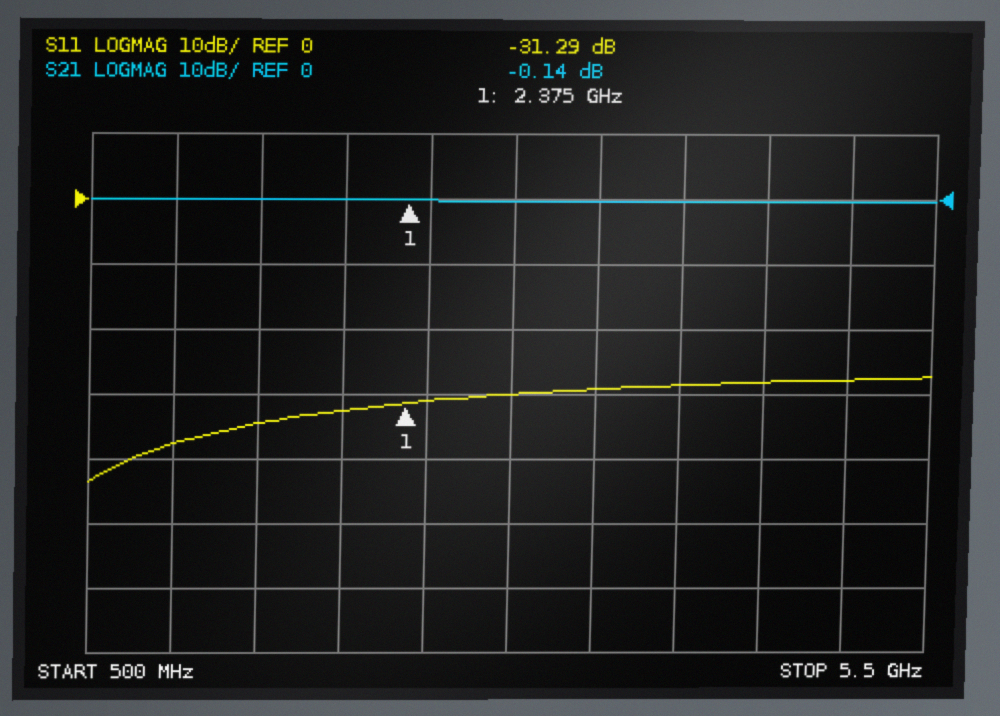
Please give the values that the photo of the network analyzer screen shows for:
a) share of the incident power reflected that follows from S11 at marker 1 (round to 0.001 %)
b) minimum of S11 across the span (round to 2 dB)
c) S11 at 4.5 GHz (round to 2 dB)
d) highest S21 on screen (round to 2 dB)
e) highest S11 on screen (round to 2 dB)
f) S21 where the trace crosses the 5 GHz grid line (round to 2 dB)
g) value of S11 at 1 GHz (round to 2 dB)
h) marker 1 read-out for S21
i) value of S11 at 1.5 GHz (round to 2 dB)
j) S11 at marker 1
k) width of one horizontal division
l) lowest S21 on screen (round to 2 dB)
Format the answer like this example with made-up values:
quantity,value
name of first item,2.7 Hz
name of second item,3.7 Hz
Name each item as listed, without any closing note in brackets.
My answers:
quantity,value
share of the incident power reflected that follows from S11 at marker 1,0.074 %
minimum of S11 across the span,-44 dB
S11 at 4.5 GHz,-28 dB
highest S21 on screen,0 dB
highest S11 on screen,-28 dB
S21 where the trace crosses the 5 GHz grid line,0 dB
value of S11 at 1 GHz,-38 dB
marker 1 read-out for S21,-0.14 dB
value of S11 at 1.5 GHz,-34 dB
S11 at marker 1,-31.29 dB
width of one horizontal division,500 MHz
lowest S21 on screen,0 dB
